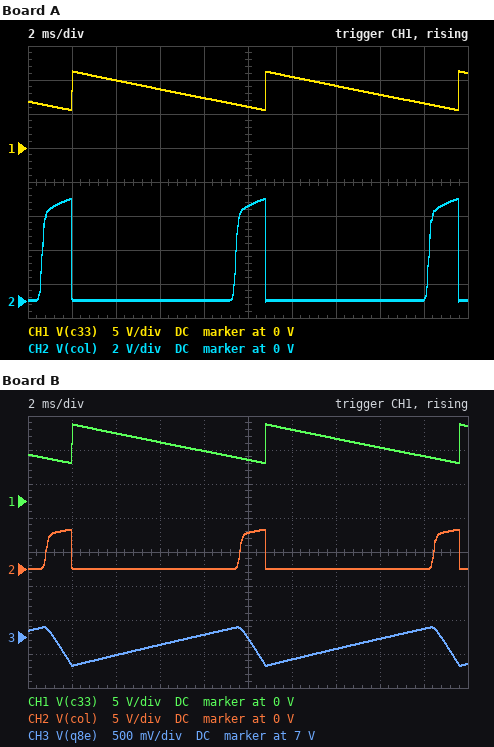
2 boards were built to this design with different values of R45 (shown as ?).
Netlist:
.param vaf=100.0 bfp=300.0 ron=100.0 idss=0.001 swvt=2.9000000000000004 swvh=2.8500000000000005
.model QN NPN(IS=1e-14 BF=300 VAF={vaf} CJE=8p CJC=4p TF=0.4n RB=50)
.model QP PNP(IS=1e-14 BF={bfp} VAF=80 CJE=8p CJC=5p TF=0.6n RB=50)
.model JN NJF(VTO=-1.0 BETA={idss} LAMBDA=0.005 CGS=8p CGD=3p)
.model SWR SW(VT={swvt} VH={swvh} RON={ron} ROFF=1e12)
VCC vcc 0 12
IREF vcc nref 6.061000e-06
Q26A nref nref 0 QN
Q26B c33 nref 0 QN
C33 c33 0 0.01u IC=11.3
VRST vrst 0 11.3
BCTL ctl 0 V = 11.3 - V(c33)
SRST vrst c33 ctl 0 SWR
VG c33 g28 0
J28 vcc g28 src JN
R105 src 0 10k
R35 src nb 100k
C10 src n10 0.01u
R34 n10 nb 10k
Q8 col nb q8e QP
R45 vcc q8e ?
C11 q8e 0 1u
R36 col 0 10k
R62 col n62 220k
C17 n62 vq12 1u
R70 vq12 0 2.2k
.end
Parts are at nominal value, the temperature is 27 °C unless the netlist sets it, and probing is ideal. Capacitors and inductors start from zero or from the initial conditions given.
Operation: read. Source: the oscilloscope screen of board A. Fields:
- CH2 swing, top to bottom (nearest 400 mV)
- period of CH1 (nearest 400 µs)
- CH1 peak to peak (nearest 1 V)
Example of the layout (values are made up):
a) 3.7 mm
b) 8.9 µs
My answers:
a) 6.0 V
b) 8.8 ms
c) 6 V
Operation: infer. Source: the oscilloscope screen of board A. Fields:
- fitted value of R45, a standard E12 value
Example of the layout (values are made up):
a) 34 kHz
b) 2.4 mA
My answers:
a) 56 kΩ
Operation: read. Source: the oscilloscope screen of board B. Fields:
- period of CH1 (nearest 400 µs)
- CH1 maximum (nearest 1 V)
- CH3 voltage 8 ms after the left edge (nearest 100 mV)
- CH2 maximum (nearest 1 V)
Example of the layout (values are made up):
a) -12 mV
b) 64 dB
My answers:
a) 8.8 ms
b) 11 V
c) 7.0 V
d) 6 V
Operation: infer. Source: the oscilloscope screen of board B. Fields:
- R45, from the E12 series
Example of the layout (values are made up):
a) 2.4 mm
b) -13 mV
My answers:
a) 68 kΩ
